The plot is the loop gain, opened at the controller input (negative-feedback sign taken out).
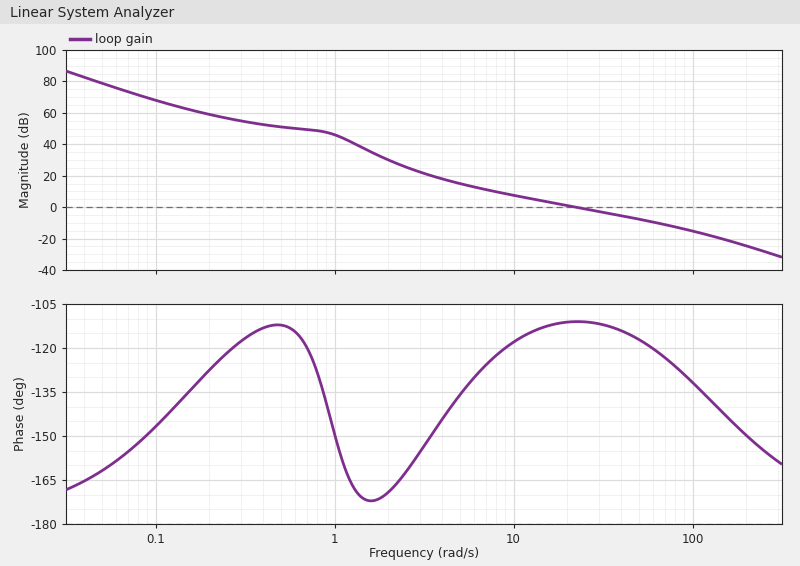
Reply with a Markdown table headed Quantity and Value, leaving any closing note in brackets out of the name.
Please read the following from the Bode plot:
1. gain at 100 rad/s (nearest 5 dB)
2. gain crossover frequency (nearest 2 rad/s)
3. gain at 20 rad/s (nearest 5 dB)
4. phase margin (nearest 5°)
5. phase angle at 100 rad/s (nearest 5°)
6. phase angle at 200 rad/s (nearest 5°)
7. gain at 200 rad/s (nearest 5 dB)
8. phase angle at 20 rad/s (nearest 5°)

| Quantity | Value |
|---|---|
| gain at 100 rad/s | -15 dB |
| gain crossover frequency | 22 rad/s |
| gain at 20 rad/s | 0 dB |
| phase margin | 70° |
| phase angle at 100 rad/s | -130° |
| phase angle at 200 rad/s | -150° |
| gain at 200 rad/s | -25 dB |
| phase angle at 20 rad/s | -110° |
